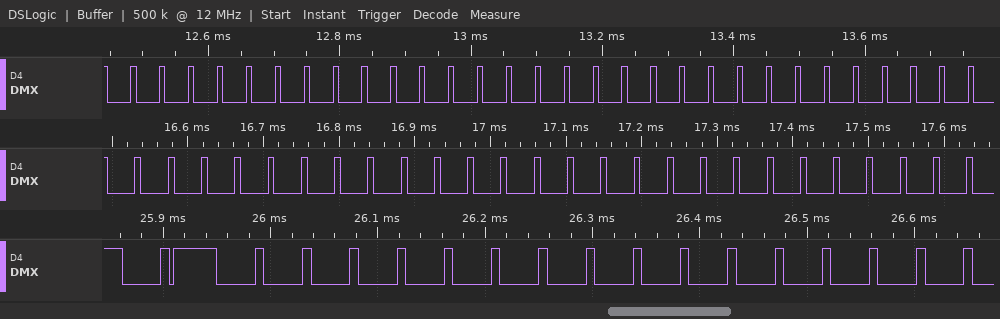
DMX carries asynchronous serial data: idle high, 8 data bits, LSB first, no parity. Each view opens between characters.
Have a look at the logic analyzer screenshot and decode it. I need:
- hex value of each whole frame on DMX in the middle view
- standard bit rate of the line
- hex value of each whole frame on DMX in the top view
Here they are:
08, 08, 08, 08, 08, 08, 08, 08, 08, 08, 08, 08, 08
115200 baud
08, 08, 08, 08, 08, 08, 08, 08, 08, 08, 08, 08, 08, 08, 08
